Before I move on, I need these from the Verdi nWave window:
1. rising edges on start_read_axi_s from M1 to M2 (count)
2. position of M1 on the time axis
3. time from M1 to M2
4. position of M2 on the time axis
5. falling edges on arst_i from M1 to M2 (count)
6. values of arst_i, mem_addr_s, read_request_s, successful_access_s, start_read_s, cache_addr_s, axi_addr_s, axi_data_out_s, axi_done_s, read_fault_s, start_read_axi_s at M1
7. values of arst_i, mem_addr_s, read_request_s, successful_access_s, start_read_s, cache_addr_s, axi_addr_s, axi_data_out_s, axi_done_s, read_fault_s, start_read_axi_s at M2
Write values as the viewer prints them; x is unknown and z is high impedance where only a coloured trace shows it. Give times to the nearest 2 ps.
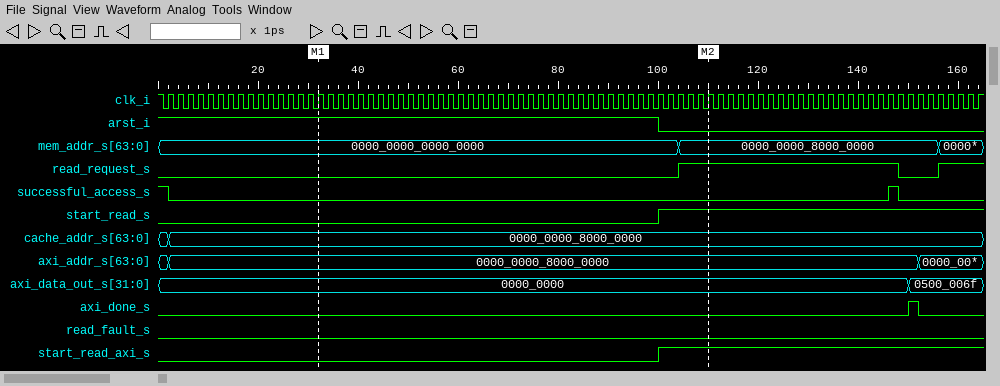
1
32 ps
78 ps
110 ps
1
arst_i=1, mem_addr_s=0000_0000_0000_0000, read_request_s=0, successful_access_s=0, start_read_s=0, cache_addr_s=0000_0000_8000_0000, axi_addr_s=0000_0000_8000_0000, axi_data_out_s=0000_0000, axi_done_s=0, read_fault_s=0, start_read_axi_s=0
arst_i=0, mem_addr_s=0000_0000_8000_0000, read_request_s=1, successful_access_s=0, start_read_s=1, cache_addr_s=0000_0000_8000_0000, axi_addr_s=0000_0000_8000_0000, axi_data_out_s=0000_0000, axi_done_s=0, read_fault_s=0, start_read_axi_s=1
